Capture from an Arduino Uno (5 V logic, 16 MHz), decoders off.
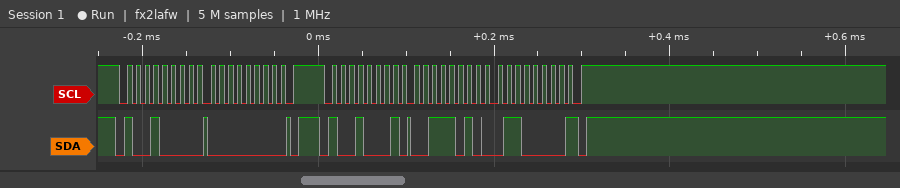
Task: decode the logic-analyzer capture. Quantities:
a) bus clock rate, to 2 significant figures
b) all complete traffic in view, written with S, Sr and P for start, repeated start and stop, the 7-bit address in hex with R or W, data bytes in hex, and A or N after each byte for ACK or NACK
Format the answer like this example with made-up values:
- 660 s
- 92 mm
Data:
- 100 kHz
- S 48W A 00 A P S 48R A 3A A 60 N P
